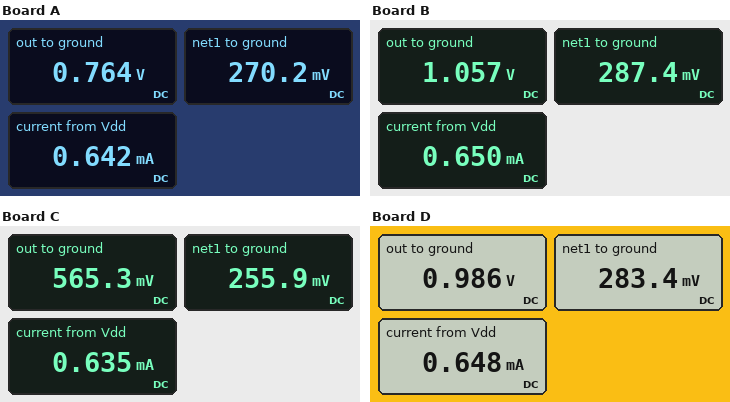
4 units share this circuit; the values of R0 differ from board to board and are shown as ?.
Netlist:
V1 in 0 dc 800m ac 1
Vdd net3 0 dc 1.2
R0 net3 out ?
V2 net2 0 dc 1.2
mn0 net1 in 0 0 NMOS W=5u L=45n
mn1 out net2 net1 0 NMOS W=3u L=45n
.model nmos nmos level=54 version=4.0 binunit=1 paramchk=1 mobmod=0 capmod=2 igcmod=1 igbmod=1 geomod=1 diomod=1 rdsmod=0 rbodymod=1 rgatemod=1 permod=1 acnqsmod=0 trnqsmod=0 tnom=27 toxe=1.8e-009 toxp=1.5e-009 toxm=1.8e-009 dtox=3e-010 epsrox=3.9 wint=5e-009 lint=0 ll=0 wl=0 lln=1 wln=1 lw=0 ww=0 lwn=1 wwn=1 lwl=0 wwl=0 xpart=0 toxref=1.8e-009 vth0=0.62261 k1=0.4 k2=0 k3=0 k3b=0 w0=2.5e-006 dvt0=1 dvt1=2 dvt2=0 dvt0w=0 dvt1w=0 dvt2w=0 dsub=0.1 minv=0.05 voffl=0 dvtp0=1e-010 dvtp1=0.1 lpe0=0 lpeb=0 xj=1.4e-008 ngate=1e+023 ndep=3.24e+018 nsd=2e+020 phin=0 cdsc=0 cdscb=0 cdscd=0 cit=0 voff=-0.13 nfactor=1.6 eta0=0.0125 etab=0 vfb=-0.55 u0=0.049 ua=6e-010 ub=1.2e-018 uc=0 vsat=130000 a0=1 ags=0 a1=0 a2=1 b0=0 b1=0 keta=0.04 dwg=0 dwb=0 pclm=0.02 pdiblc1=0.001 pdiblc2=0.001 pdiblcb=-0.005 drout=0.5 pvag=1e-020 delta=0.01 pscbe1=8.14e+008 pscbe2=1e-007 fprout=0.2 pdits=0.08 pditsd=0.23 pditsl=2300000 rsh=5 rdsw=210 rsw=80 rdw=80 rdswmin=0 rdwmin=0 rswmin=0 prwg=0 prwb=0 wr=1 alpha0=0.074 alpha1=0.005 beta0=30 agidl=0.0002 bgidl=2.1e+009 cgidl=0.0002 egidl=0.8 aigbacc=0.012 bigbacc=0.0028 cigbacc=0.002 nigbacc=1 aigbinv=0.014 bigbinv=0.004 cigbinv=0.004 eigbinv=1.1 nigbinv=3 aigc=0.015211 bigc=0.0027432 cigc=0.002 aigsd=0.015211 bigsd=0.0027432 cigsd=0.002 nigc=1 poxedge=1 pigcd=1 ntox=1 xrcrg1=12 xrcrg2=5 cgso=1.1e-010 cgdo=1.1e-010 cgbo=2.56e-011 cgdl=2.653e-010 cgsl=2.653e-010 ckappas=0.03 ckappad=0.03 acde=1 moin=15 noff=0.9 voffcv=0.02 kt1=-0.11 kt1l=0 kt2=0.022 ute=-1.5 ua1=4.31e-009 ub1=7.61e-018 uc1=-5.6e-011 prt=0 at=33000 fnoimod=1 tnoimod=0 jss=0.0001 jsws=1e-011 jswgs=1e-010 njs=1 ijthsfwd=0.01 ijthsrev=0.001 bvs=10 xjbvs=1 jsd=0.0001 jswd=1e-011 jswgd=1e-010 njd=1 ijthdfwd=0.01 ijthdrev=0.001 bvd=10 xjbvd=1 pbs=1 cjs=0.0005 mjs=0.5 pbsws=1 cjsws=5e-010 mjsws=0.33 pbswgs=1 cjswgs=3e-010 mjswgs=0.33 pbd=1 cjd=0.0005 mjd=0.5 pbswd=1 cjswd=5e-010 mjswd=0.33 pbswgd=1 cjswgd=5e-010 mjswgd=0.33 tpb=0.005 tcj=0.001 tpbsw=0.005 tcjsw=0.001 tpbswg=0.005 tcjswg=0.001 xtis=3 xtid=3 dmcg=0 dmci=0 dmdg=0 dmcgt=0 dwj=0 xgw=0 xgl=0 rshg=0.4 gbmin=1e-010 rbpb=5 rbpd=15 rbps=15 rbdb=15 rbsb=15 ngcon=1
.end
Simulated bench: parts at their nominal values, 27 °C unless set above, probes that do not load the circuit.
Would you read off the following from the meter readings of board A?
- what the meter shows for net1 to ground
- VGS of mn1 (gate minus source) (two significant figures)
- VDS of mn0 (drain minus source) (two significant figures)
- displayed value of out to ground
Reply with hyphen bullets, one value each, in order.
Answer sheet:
- 270.2 mV
- 930 mV
- 270 mV
- 0.764 V
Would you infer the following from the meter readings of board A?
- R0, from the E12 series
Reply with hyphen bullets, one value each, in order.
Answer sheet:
- 680 Ω
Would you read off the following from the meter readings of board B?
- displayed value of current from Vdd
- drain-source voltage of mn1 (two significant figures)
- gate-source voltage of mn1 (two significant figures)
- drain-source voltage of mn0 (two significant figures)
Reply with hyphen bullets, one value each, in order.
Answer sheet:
- 0.650 mA
- 770 mV
- 910 mV
- 290 mV
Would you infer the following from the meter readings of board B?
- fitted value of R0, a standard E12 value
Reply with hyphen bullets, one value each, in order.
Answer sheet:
- 220 Ω
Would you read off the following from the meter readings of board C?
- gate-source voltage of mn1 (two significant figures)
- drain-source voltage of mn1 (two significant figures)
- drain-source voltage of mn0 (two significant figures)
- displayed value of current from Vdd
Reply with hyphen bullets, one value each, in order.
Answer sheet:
- 940 mV
- 310 mV
- 260 mV
- 0.635 mA
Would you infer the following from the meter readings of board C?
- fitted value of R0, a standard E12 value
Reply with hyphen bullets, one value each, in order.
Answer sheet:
- 1 kΩ
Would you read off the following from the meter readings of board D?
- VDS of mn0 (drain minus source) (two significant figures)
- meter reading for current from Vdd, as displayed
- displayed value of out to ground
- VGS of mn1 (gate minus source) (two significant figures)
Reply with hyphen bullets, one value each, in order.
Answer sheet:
- 280 mV
- 0.648 mA
- 0.986 V
- 920 mV
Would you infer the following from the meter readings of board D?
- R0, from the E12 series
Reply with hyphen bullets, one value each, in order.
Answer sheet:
- 330 Ω
